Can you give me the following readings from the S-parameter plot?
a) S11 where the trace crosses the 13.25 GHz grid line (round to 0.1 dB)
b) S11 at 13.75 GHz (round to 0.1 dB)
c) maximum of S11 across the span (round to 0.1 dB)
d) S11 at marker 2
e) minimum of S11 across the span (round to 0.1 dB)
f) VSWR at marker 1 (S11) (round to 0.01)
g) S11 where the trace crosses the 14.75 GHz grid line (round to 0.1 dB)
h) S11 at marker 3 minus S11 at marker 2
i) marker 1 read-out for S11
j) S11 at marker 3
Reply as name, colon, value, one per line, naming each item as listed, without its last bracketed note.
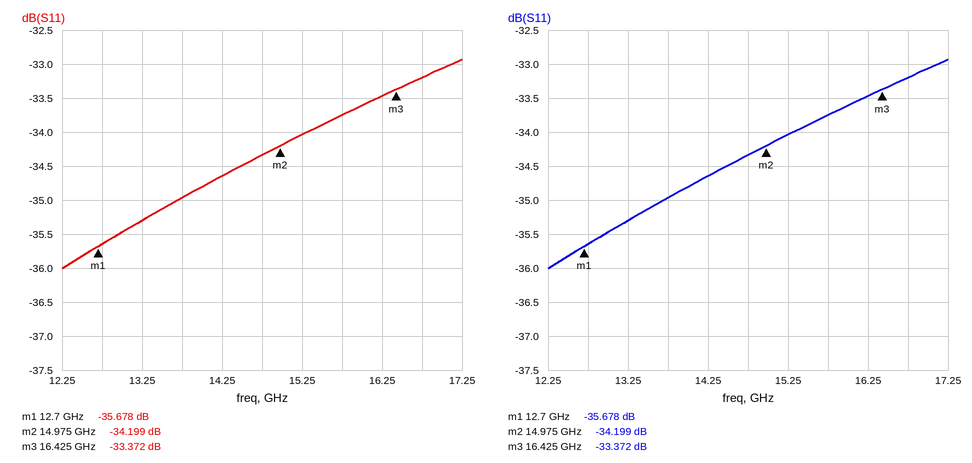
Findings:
S11 where the trace crosses the 13.25 GHz grid line: -35.3 dB
S11 at 13.75 GHz: -35.0 dB
maximum of S11 across the span: -32.9 dB
S11 at marker 2: -34.199 dB
minimum of S11 across the span: -36.0 dB
VSWR at marker 1 (S11): 1.03
S11 where the trace crosses the 14.75 GHz grid line: -34.3 dB
S11 at marker 3 minus S11 at marker 2: 0.827 dB
marker 1 read-out for S11: -35.678 dB
S11 at marker 3: -33.372 dB
